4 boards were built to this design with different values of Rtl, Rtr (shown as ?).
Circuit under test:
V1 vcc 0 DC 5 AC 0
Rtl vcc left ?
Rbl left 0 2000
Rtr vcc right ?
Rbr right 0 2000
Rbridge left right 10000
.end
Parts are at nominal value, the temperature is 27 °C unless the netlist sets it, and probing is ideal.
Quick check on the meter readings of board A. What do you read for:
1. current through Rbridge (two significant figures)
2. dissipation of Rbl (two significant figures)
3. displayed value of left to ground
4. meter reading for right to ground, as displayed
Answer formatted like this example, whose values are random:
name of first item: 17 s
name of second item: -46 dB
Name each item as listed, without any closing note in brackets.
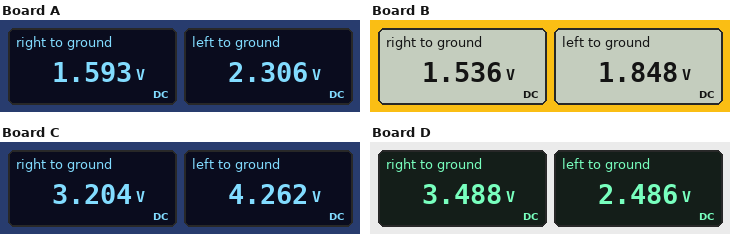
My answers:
current through Rbridge: 71 µA
dissipation of Rbl: 2.7 mW
displayed value of left to ground: 2.306 V
meter reading for right to ground, as displayed: 1.593 V
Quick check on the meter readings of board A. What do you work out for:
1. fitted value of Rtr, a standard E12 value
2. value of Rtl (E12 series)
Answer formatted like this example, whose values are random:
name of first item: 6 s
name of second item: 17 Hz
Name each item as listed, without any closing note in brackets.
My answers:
fitted value of Rtr, a standard E12 value: 4.7 kΩ
value of Rtl: 2.2 kΩ
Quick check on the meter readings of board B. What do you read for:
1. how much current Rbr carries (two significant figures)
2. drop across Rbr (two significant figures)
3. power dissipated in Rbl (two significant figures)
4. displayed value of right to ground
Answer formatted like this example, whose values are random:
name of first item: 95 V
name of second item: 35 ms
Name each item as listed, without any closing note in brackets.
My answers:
how much current Rbr carries: 770 µA
drop across Rbr: 1.5 V
power dissipated in Rbl: 1.7 mW
displayed value of right to ground: 1.536 V
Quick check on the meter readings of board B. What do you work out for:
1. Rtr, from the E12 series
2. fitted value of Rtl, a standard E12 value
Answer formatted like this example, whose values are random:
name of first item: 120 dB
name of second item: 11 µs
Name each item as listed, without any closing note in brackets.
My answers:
Rtr, from the E12 series: 4.7 kΩ
fitted value of Rtl, a standard E12 value: 3.3 kΩ
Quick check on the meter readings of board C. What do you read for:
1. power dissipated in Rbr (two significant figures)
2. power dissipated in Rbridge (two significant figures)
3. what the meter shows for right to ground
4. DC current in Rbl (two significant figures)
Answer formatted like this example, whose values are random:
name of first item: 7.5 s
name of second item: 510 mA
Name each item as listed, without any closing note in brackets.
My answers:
power dissipated in Rbr: 5.1 mW
power dissipated in Rbridge: 110 µW
what the meter shows for right to ground: 3.204 V
DC current in Rbl: 2.1 mA
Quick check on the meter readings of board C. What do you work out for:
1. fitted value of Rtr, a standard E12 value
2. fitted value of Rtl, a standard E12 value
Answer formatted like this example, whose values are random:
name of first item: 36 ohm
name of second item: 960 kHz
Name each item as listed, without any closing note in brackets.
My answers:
fitted value of Rtr, a standard E12 value: 1.2 kΩ
fitted value of Rtl, a standard E12 value: 330 Ω
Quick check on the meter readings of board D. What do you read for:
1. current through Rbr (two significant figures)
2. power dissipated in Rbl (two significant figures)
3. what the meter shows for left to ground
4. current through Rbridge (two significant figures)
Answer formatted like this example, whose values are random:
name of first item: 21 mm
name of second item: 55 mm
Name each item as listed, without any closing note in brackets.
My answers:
current through Rbr: 1.7 mA
power dissipated in Rbl: 3.1 mW
what the meter shows for left to ground: 2.486 V
current through Rbridge: 100 µA
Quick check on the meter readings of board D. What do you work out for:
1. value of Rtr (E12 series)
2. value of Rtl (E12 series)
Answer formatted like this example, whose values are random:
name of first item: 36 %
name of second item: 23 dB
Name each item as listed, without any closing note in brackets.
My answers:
value of Rtr: 820 Ω
value of Rtl: 2.2 kΩ
